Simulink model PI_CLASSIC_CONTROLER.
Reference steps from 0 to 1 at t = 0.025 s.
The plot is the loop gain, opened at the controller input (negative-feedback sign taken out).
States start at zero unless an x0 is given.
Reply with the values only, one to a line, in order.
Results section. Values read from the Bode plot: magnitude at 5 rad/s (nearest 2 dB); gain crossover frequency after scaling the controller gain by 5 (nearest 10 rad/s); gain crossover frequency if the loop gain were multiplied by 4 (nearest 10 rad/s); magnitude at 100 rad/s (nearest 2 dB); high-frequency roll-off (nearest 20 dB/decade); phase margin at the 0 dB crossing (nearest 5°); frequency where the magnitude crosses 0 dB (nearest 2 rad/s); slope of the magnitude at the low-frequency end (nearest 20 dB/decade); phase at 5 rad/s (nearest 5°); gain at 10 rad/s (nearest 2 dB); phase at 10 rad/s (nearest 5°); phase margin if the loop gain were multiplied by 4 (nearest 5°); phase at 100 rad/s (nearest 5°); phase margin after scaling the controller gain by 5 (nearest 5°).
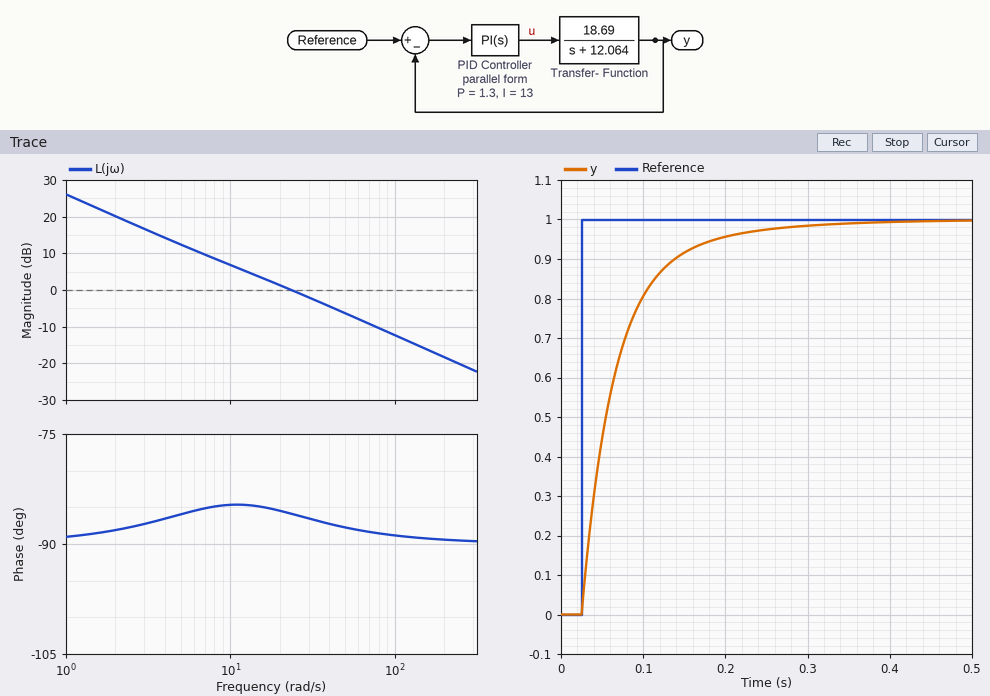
12 dB
120 rad/s
100 rad/s
-12 dB
-20 dB/decade
95°
24 rad/s
-20 dB/decade
-85°
6 dB
-85°
90°
-90°
90°
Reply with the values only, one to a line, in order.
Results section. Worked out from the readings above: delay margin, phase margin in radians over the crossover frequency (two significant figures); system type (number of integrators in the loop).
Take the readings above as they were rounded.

0.069 s
1
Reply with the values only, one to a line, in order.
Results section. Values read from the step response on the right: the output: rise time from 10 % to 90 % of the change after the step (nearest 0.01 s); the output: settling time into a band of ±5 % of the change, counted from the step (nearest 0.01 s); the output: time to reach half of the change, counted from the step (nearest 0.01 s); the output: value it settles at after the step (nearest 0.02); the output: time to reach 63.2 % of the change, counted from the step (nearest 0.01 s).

0.11 s
0.16 s
0.03 s
1.00
0.04 s
